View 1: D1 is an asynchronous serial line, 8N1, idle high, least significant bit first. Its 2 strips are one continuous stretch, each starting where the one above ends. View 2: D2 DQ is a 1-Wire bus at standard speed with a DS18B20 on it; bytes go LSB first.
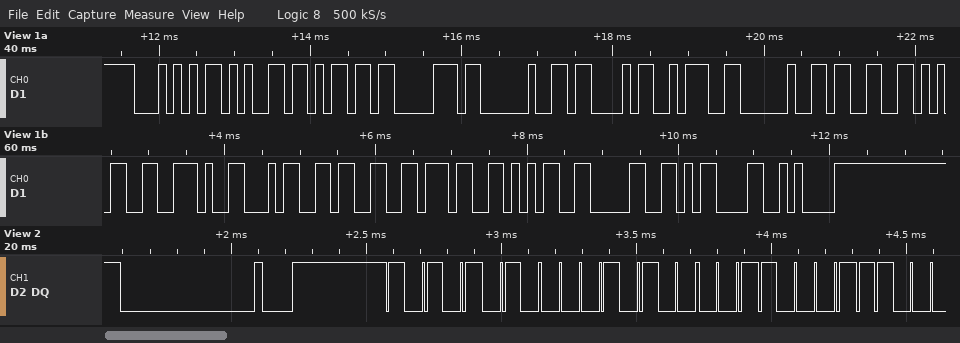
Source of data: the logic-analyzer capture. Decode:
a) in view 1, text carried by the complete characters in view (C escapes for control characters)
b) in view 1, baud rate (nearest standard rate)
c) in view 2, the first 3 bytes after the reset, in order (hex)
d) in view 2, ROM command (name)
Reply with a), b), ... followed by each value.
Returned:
a) "Temp C: 35.43750\r\n"
b) 9600 baud
c) 55 28 8C
d) Match ROM
